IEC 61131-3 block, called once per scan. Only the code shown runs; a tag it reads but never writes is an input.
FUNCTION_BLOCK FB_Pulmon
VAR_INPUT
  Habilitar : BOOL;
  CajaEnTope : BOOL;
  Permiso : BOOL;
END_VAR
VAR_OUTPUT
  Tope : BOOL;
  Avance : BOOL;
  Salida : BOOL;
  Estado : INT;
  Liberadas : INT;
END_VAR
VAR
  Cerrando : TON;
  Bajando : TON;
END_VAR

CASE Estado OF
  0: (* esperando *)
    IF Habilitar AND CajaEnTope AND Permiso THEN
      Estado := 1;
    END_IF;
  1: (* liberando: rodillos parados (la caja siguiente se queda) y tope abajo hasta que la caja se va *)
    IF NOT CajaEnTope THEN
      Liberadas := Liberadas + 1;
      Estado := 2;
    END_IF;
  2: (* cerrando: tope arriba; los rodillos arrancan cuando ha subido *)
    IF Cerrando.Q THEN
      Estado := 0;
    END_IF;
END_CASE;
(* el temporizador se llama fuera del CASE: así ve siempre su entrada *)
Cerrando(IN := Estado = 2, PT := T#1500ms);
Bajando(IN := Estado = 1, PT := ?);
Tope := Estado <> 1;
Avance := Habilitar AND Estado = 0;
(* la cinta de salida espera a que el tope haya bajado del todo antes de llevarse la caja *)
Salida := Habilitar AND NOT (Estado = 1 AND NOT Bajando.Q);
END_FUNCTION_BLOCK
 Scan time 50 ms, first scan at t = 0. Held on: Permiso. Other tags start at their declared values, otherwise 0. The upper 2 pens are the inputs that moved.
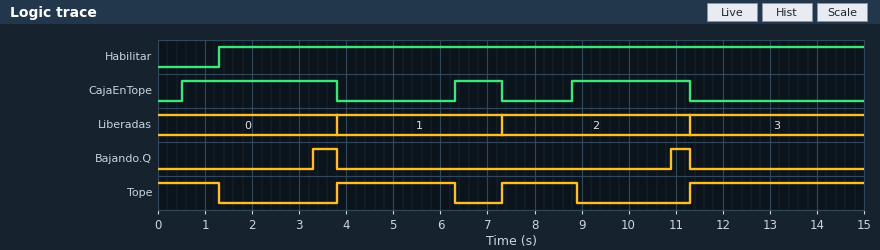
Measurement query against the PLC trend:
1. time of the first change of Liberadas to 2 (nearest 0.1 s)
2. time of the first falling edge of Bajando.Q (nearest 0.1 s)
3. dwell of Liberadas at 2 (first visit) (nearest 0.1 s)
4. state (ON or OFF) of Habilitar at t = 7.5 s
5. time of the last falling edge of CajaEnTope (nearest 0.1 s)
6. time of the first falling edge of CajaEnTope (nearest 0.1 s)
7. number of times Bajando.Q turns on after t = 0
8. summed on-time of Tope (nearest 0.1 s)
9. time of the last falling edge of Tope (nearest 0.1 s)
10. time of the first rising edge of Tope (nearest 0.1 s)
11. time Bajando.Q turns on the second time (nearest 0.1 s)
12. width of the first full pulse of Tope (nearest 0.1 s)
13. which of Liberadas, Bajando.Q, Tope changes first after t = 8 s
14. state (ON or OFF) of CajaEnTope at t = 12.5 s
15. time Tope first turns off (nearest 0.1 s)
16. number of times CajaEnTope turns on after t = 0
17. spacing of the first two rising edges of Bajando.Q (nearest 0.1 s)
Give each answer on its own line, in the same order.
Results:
7.3 s
3.8 s
4.0 s
ON
11.3 s
3.8 s
2
9.1 s
8.9 s
3.8 s
10.9 s
2.5 s
Tope
OFF
1.3 s
3
7.6 s
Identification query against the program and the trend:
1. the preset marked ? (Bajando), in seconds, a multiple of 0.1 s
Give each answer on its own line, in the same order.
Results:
2.0 s
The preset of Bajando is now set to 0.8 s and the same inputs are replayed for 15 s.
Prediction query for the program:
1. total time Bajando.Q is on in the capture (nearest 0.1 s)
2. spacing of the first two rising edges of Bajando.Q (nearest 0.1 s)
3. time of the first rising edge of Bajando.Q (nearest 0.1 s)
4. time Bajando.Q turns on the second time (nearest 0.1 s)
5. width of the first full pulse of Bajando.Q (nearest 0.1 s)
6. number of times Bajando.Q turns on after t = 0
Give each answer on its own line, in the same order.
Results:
3.5 s
5.0 s
2.1 s
7.1 s
1.7 s
3
